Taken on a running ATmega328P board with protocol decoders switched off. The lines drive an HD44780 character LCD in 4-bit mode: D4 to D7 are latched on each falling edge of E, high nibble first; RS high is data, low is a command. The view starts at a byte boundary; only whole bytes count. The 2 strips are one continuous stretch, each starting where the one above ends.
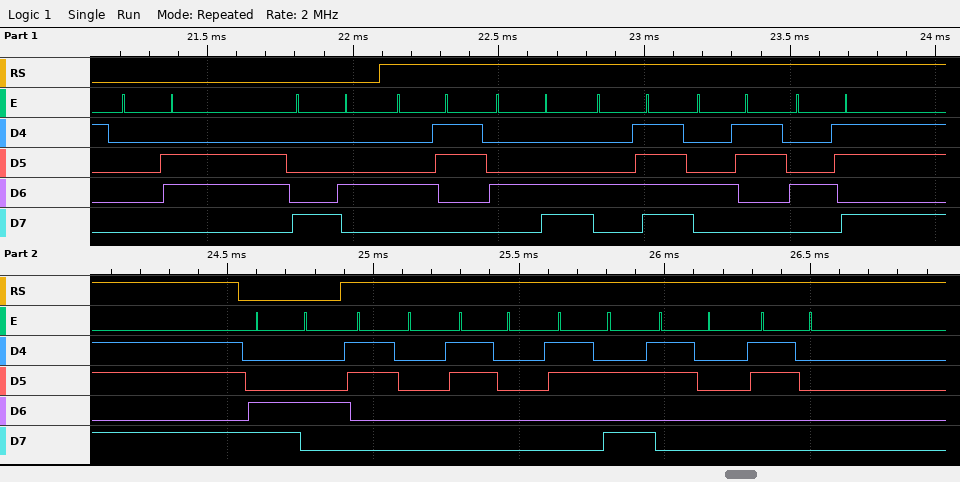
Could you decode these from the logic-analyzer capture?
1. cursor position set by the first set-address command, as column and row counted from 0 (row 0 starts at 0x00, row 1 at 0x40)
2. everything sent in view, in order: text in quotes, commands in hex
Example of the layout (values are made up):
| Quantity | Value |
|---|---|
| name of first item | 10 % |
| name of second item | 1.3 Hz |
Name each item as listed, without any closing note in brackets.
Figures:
| Quantity | Value |
|---|---|
| cursor position set by the first set-address command, as column and row counted from 0 | column 4, row 0 |
| everything sent in view, in order: text in quotes, commands in hex | 0x06 0x84 "CLOCK" 0xC4 "00:00" |
